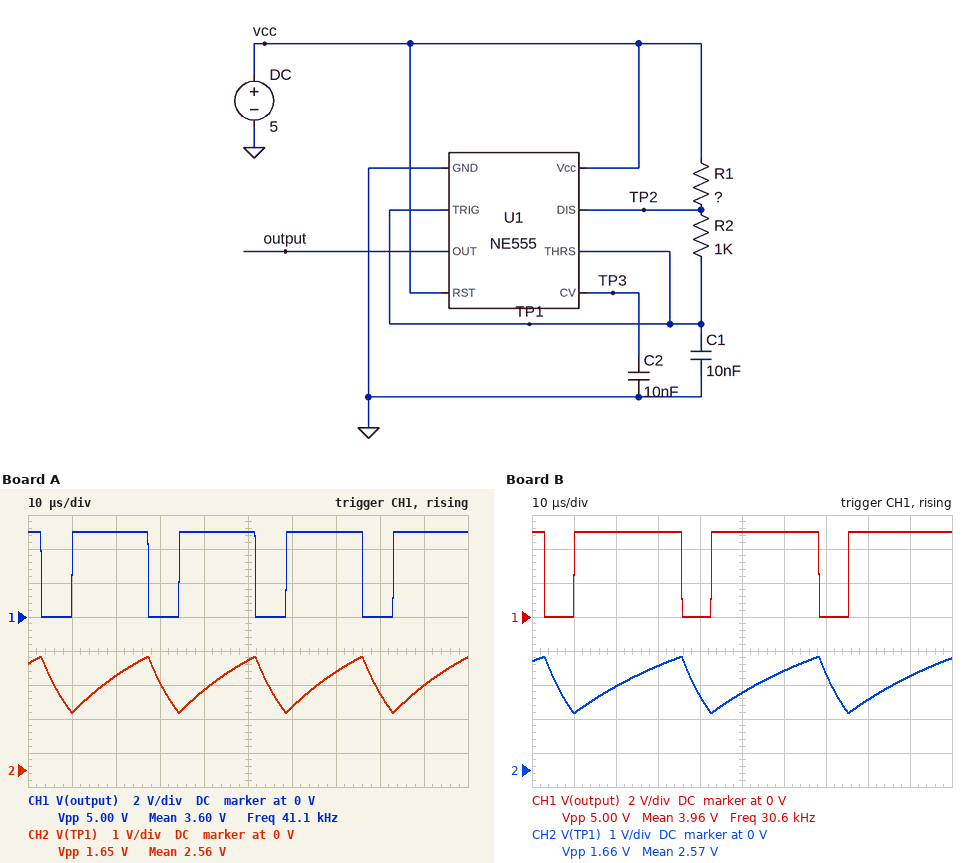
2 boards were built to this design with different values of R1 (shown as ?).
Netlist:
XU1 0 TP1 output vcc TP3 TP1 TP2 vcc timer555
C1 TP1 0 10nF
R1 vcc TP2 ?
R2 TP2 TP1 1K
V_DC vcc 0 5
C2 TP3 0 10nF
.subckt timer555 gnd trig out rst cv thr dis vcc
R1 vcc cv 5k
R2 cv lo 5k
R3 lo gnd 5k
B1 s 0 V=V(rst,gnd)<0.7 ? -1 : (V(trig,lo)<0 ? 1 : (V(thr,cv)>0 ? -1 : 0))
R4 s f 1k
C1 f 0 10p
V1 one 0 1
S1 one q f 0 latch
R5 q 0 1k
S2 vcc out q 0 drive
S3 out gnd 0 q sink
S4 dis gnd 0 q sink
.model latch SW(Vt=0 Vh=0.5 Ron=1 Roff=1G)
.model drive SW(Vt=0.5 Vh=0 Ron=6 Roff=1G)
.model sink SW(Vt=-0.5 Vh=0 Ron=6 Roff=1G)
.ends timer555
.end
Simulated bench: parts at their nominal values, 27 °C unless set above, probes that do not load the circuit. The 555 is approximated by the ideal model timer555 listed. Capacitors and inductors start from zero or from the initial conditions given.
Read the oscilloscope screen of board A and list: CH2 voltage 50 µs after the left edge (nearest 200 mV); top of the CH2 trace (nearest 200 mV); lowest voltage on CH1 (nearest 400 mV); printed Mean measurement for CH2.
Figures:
3.2 V
3.4 V
0 V
2.56 V
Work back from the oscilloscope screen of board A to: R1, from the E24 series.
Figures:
1.5 kΩ
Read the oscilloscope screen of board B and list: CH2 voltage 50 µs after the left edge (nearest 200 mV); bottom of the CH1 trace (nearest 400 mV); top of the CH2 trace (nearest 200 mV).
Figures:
2.2 V
0 V
3.4 V
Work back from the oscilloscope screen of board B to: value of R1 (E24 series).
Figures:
2.7 kΩ
